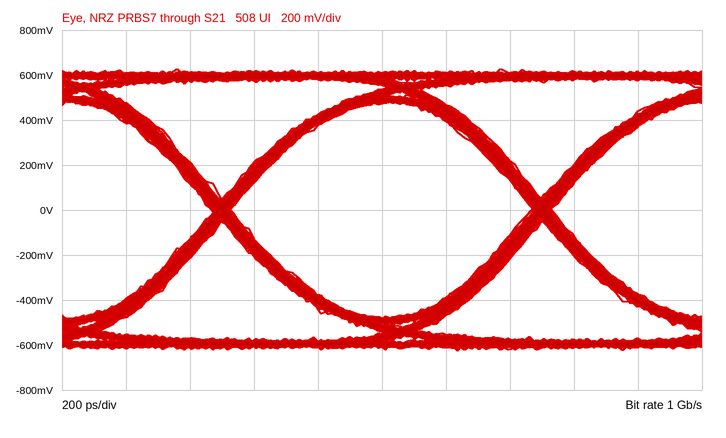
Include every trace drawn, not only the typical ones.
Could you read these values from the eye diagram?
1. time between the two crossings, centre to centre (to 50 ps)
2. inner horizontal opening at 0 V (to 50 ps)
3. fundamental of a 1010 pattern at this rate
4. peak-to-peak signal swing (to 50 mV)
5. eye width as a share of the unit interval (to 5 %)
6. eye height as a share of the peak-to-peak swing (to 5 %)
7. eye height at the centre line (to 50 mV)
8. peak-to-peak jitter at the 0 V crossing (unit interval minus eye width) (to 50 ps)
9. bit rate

1.00 ns
950 ps
500 MHz
1.25 V
95 %
75 %
950 mV
50 ps
1 Gb/s
